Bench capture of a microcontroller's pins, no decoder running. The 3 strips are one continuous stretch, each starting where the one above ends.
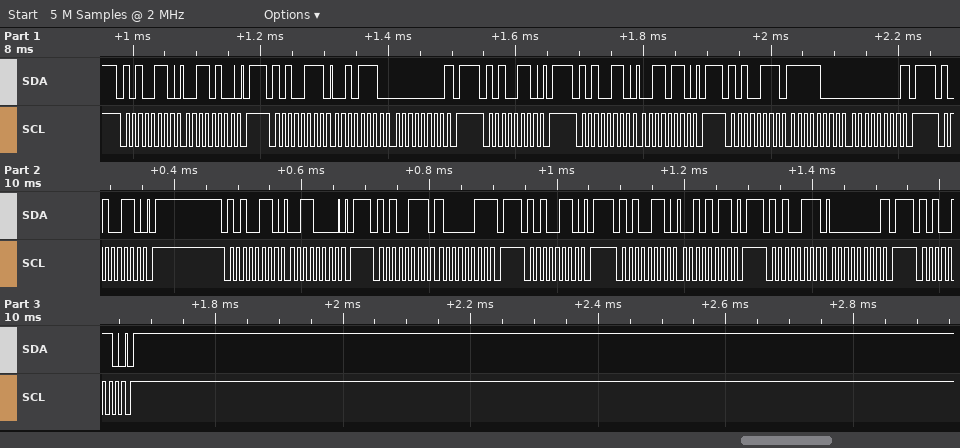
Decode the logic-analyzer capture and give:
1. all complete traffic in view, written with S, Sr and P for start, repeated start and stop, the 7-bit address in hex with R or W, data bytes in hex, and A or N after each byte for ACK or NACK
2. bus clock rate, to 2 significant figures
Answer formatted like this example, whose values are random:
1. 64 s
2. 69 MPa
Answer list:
1. S 53W A 34 A P S 53R A 2E A 00 N P S 53W A P S 53W A 36 A P S 53R A F8 A 00 N P S 53W A P S 53W A 30 A P S 53R A 83 N P S 53W A P S 53W A 2B A P S 53R A 00 N P S 53W A P
2. 100 kHz
